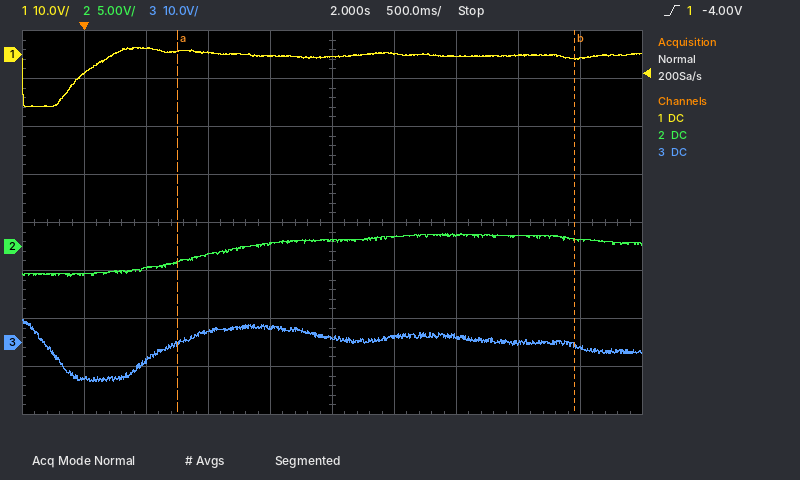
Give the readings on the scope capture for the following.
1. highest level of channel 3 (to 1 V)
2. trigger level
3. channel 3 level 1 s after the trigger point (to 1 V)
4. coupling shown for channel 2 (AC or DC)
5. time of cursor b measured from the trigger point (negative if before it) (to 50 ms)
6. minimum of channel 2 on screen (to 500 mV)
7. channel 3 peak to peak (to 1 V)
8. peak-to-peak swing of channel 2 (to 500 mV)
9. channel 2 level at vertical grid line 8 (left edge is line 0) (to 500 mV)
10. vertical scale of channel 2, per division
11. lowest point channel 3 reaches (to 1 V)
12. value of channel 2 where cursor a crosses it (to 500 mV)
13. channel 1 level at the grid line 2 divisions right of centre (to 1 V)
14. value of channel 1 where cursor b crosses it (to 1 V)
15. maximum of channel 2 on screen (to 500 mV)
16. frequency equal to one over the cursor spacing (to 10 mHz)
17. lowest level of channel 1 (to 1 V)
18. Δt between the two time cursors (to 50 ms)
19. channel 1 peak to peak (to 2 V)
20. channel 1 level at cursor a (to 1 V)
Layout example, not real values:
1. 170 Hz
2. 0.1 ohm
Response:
1. 5 V
2. -4.00 V
3. 2 V
4. DC
5. +3.95 s
6. -3.0 V
7. 13 V
8. 4.5 V
9. 1.0 V
10. 5 V
11. -8 V
12. -1.5 V
13. 0 V
14. -1 V
15. 1.5 V
16. 310 mHz
17. -11 V
18. 3.20 s
19. 12 V
20. 1 V
